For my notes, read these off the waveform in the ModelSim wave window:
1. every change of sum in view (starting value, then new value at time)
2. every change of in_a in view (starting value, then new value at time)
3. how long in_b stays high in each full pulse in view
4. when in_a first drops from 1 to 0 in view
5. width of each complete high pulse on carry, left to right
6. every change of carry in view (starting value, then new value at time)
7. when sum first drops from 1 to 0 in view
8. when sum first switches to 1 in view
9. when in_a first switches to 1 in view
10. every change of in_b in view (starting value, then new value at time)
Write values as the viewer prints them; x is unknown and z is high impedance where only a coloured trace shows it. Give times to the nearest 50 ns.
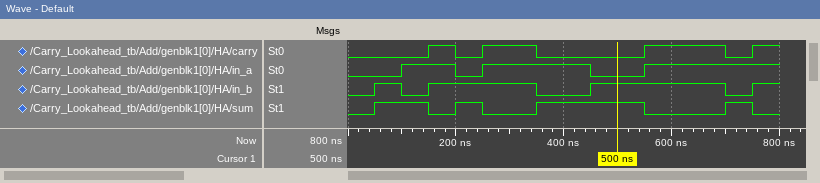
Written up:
0, 1 at 50 ns, 0 at 150 ns, 1 at 200 ns, 0 at 250 ns, 1 at 350 ns, 0 at 550 ns, 1 at 700 ns, 0 at 750 ns
0, 1 at 100 ns, 0 at 200 ns, 1 at 250 ns, 0 at 450 ns, 1 at 550 ns
50 ns, 200 ns, 250 ns
200 ns
50 ns, 100 ns, 150 ns
0, 1 at 150 ns, 0 at 200 ns, 1 at 250 ns, 0 at 350 ns, 1 at 550 ns, 0 at 700 ns, 1 at 750 ns
150 ns
50 ns
100 ns
0, 1 at 50 ns, 0 at 100 ns, 1 at 150 ns, 0 at 350 ns, 1 at 450 ns, 0 at 700 ns, 1 at 750 ns
